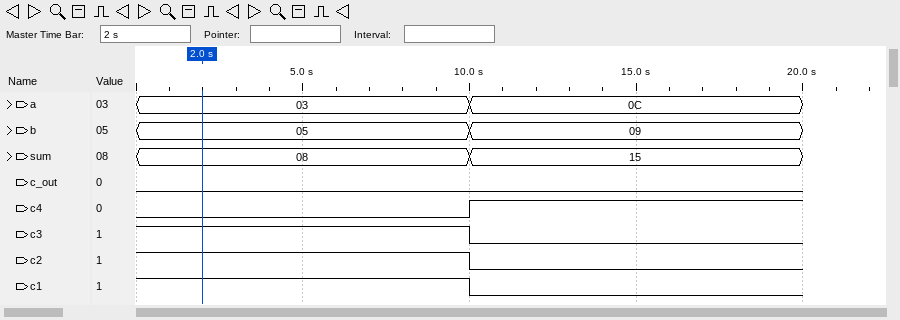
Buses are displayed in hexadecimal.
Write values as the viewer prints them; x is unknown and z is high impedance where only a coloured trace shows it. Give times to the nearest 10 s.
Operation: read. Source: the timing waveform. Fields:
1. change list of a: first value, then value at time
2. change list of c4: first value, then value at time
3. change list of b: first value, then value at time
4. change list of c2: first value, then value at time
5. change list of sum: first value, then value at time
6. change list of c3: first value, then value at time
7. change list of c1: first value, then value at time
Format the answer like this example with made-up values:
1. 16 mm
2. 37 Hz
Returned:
1. 03, 0C at 10 s
2. 0, 1 at 10 s
3. 05, 09 at 10 s
4. 1, 0 at 10 s
5. 08, 15 at 10 s
6. 1, 0 at 10 s
7. 1, 0 at 10 s
